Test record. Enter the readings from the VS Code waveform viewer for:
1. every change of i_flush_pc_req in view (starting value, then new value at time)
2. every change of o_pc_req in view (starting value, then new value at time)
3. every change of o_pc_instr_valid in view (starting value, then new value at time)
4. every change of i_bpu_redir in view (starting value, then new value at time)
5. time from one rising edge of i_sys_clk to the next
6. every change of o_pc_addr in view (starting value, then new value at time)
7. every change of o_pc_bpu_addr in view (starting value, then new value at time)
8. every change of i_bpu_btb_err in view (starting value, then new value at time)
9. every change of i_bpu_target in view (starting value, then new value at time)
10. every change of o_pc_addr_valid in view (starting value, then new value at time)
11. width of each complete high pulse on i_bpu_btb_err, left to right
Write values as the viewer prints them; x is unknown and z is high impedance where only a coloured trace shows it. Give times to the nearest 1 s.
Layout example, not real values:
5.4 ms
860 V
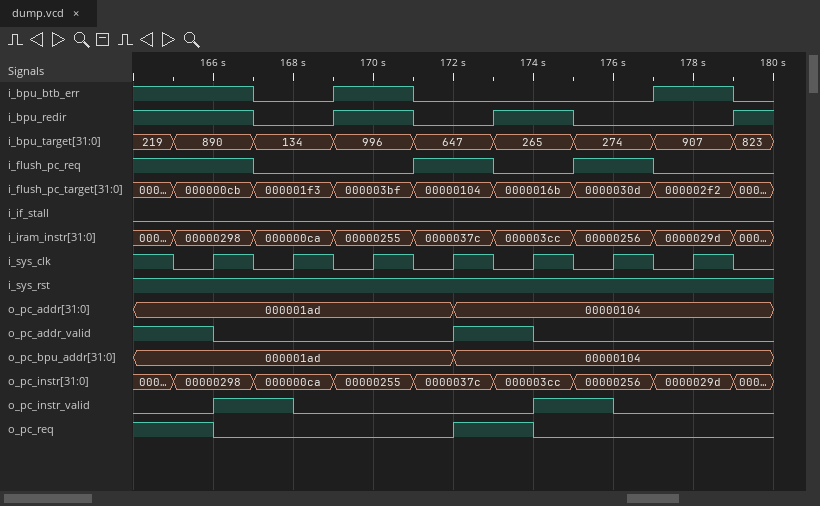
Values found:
1, 0 at 167 s, 1 at 171 s, 0 at 173 s, 1 at 175 s, 0 at 177 s
1, 0 at 166 s, 1 at 172 s, 0 at 174 s
0, 1 at 166 s, 0 at 168 s, 1 at 174 s, 0 at 176 s
1, 0 at 167 s, 1 at 169 s, 0 at 171 s, 1 at 173 s, 0 at 175 s, 1 at 179 s
2 s
000001ad, 00000104 at 172 s
000001ad, 00000104 at 172 s
1, 0 at 167 s, 1 at 169 s, 0 at 171 s, 1 at 177 s, 0 at 179 s
219, 890 at 165 s, 134 at 167 s, 996 at 169 s, 647 at 171 s, 265 at 173 s, 274 at 175 s, 907 at 177 s, 823 at 179 s
1, 0 at 166 s, 1 at 172 s, 0 at 174 s
2 s, 2 s
